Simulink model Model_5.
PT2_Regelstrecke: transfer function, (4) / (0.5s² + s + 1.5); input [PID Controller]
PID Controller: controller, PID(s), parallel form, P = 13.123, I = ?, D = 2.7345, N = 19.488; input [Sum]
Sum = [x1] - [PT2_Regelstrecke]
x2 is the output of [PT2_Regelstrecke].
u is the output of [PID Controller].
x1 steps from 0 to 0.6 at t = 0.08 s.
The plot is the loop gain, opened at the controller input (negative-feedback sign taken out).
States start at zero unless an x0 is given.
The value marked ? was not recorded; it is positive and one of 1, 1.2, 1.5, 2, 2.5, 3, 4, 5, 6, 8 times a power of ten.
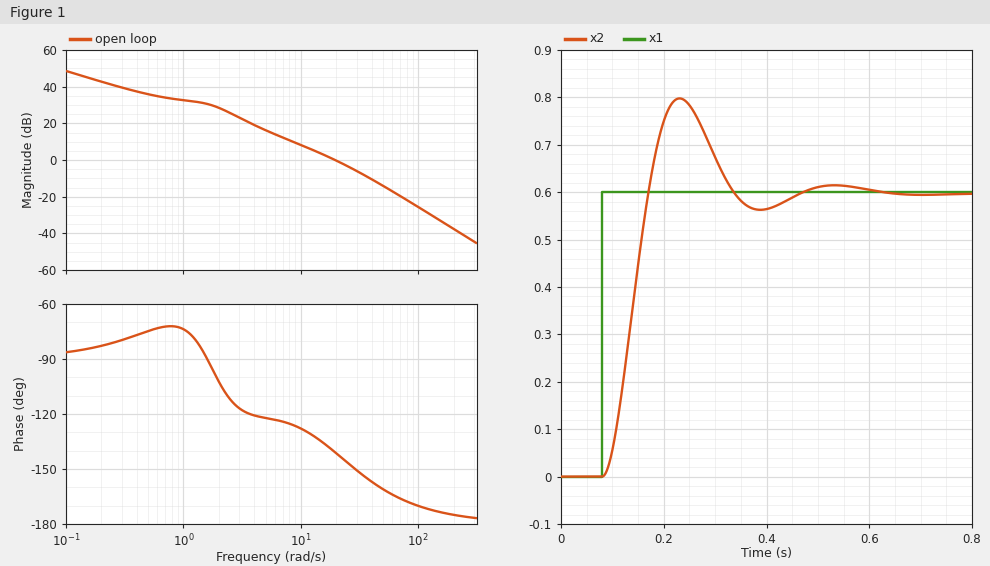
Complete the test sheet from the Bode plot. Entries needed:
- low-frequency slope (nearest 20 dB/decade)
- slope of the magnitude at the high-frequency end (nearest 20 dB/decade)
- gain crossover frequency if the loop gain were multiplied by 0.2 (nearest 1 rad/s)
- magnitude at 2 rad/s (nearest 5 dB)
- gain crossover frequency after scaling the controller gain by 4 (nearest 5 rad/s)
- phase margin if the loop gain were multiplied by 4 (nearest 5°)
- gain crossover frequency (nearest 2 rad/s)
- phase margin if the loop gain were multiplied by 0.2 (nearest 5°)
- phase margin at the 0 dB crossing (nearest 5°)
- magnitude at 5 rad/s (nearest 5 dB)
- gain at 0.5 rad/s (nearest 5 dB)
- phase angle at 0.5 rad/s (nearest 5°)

-20 dB/decade
-40 dB/decade
6 rad/s
30 dB
45 rad/s
20°
20 rad/s
55°
40°
15 dB
35 dB
-75°
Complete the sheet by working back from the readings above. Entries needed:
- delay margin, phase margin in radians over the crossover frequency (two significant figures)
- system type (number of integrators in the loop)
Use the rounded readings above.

0.035 s
1
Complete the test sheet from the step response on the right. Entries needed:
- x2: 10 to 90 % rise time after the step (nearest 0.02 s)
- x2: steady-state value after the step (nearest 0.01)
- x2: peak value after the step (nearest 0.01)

0.06 s
0.60
0.80
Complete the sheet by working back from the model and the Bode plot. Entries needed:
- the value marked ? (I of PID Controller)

10
